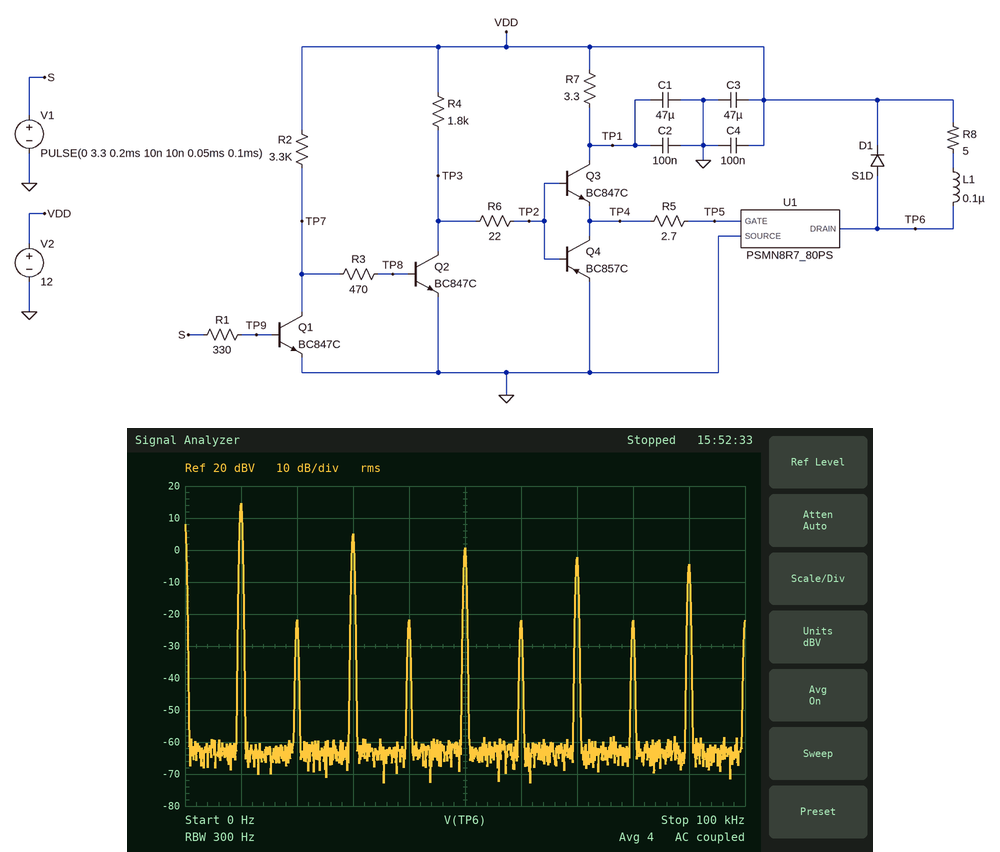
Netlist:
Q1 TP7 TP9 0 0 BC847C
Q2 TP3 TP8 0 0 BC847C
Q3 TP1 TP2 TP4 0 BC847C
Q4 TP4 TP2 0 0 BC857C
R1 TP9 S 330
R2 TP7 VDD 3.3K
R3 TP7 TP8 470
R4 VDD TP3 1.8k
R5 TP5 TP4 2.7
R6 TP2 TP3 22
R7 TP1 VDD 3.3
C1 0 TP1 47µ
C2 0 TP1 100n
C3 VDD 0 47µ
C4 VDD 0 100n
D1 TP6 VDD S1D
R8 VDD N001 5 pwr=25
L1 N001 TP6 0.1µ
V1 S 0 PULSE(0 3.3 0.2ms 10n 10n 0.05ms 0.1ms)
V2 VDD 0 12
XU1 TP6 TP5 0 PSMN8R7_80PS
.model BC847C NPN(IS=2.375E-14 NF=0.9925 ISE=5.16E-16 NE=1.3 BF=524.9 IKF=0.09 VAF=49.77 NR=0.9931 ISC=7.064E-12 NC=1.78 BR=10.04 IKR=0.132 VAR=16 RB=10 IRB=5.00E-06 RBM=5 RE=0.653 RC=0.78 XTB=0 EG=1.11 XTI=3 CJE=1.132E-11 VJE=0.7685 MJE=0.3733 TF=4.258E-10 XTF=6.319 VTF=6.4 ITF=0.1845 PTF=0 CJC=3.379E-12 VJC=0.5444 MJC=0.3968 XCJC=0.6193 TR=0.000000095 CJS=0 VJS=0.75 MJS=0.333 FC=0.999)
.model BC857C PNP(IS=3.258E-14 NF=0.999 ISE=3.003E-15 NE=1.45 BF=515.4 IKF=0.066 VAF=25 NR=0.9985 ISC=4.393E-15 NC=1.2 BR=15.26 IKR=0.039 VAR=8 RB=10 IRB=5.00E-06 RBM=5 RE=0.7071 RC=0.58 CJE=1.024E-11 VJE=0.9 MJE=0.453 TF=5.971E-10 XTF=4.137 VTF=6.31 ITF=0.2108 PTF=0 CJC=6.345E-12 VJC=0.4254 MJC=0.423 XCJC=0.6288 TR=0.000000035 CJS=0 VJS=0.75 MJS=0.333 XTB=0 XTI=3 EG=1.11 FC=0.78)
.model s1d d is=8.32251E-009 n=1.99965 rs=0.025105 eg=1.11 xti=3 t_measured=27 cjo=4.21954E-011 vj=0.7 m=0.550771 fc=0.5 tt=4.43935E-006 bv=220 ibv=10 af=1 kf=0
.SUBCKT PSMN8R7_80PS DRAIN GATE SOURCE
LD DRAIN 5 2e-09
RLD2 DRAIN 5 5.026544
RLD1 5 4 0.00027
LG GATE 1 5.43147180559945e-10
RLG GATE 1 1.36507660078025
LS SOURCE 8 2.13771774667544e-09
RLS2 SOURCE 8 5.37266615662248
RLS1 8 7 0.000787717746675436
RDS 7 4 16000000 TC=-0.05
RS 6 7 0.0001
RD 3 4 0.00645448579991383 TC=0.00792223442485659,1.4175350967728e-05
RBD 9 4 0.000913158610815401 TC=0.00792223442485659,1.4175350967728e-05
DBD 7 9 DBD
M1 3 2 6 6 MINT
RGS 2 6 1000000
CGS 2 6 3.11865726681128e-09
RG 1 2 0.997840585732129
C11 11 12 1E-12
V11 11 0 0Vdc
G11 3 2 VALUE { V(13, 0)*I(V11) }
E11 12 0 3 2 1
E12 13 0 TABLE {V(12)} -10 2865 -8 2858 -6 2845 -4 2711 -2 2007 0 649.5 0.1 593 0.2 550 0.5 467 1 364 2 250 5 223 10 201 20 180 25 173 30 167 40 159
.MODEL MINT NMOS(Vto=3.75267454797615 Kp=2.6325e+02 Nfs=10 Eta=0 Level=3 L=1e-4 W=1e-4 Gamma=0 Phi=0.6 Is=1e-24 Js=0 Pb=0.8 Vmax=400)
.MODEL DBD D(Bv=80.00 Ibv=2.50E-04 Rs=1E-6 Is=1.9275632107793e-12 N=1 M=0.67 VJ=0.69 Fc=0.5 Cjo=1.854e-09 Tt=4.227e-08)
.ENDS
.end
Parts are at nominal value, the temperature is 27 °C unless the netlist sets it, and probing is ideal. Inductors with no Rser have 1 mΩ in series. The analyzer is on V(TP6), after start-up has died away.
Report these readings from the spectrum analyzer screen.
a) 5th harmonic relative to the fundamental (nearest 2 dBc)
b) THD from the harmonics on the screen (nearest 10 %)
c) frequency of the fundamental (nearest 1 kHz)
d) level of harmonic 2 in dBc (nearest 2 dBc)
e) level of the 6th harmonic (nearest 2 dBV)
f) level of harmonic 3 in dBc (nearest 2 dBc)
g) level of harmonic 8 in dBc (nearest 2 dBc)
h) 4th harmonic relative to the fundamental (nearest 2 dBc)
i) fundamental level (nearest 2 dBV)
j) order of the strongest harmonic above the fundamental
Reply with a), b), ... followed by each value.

a) -14 dBc
b) 40 %
c) 10 kHz
d) -36 dBc
e) -22 dBV
f) -10 dBc
g) -36 dBc
h) -36 dBc
i) 14 dBV
j) 3
